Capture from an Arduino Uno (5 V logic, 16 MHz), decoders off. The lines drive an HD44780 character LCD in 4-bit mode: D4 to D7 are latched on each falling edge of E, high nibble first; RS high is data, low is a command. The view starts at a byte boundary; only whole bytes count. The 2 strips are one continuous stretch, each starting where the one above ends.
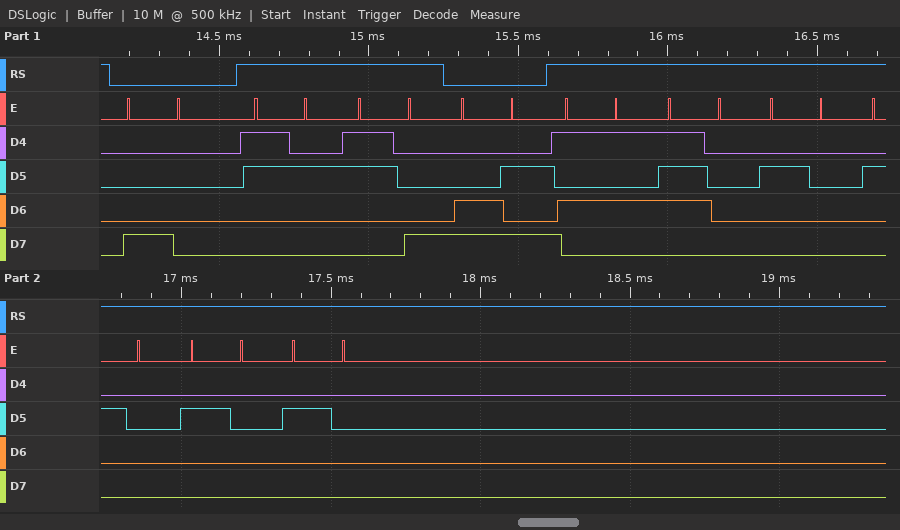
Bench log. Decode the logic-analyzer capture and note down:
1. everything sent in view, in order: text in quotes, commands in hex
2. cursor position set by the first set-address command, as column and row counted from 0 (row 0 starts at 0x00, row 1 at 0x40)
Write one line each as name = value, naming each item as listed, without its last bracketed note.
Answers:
everything sent in view, in order: text in quotes, commands in hex = 0x80 "28" 0xCA "Up    "
cursor position set by the first set-address command, as column and row counted from 0 = column 0, row 0
